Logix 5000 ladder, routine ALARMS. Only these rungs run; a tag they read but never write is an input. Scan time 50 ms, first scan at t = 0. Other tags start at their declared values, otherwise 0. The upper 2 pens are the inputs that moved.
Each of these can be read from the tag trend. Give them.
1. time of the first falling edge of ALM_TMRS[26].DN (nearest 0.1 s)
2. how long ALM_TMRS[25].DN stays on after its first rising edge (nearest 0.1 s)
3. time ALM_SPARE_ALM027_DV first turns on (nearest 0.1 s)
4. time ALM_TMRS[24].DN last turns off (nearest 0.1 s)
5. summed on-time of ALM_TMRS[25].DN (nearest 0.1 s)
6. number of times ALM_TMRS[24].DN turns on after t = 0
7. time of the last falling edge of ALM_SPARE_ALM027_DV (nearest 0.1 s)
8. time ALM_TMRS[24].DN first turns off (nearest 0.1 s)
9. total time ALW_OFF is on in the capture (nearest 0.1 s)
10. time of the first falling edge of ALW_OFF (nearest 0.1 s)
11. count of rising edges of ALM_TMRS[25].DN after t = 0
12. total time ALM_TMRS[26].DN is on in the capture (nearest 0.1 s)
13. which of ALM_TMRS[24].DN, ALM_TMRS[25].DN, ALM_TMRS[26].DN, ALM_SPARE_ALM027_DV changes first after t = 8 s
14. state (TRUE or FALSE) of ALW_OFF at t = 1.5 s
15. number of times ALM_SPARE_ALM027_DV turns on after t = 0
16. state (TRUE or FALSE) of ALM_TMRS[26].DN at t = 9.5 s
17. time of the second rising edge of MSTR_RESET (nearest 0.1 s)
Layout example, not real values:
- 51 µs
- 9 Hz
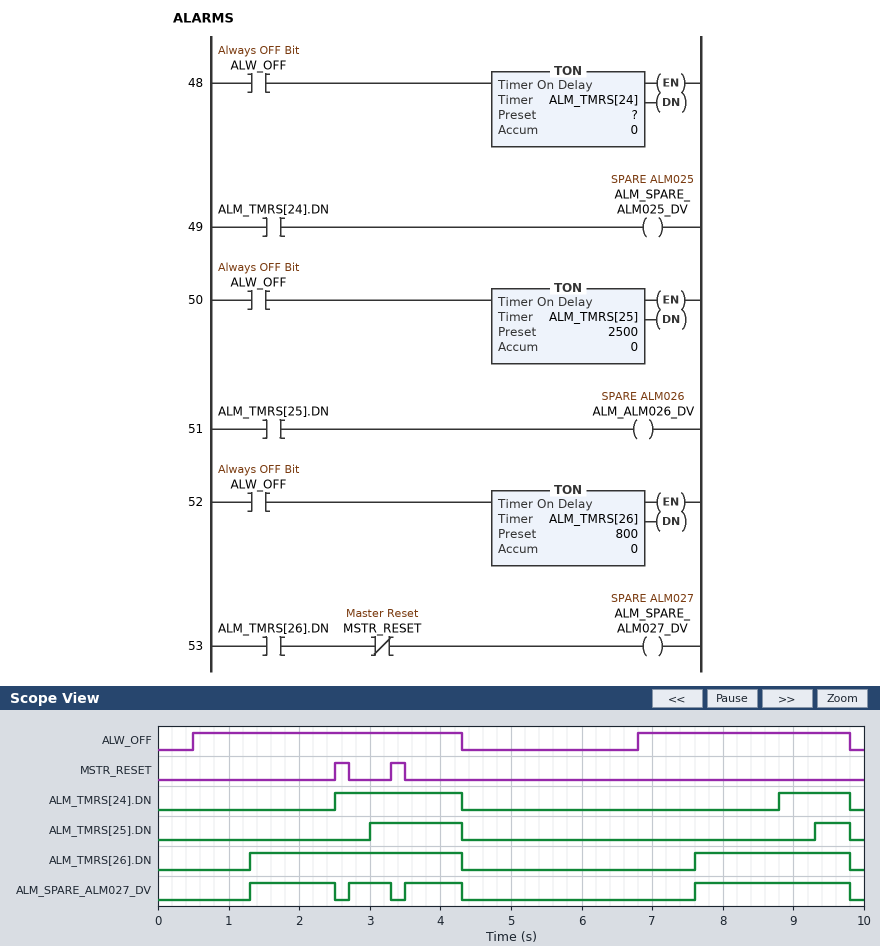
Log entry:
- 4.3 s
- 1.3 s
- 1.3 s
- 9.8 s
- 1.8 s
- 2
- 9.8 s
- 4.3 s
- 6.8 s
- 4.3 s
- 2
- 5.2 s
- ALM_TMRS[24].DN
- TRUE
- 4
- TRUE
- 3.3 s
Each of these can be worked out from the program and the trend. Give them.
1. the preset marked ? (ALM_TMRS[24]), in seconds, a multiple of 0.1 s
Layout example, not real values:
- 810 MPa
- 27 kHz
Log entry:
- 2.0 s
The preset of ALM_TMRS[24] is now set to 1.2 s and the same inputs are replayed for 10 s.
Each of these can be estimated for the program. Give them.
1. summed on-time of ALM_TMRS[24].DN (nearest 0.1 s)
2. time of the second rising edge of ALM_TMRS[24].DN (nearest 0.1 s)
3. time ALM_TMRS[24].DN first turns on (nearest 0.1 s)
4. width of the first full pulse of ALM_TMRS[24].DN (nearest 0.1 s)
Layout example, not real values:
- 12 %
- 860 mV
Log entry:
- 4.4 s
- 8.0 s
- 1.7 s
- 2.6 s
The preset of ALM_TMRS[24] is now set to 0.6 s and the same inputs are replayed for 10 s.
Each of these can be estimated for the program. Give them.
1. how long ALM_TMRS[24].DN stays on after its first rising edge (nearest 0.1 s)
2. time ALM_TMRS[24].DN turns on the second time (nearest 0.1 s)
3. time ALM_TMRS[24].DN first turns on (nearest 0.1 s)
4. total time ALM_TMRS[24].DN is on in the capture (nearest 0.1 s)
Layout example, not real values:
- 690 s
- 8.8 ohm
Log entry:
- 3.2 s
- 7.4 s
- 1.1 s
- 5.6 s
